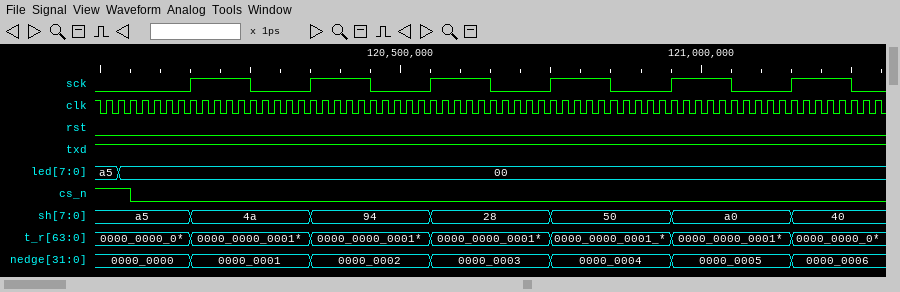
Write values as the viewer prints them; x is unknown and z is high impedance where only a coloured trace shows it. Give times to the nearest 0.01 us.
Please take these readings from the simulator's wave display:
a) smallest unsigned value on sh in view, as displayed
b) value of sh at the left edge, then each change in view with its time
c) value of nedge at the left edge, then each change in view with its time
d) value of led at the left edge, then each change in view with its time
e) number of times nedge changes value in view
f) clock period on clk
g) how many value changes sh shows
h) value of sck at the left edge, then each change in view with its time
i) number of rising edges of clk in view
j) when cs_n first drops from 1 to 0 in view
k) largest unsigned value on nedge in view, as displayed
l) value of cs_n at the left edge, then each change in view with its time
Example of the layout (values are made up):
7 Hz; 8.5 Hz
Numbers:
28; a5, 4a at 120.15 us, 94 at 120.35 us, 28 at 120.55 us, 50 at 120.75 us, a0 at 120.95 us, 40 at 121.15 us; 0000_0000, 0000_0001 at 120.15 us, 0000_0002 at 120.35 us, 0000_0003 at 120.55 us, 0000_0004 at 120.75 us, 0000_0005 at 120.95 us, 0000_0006 at 121.15 us; a5, 00 at 120.03 us; 6; 0.02 us; 6; 0, 1 at 120.15 us, 0 at 120.25 us, 1 at 120.35 us, 0 at 120.45 us, 1 at 120.55 us, 0 at 120.65 us, 1 at 120.75 us, 0 at 120.85 us, 1 at 120.95 us, 0 at 121.05 us, 1 at 121.15 us, 0 at 121.25 us; 65; 120.05 us; 0000_0006; 1, 0 at 120.05 us
